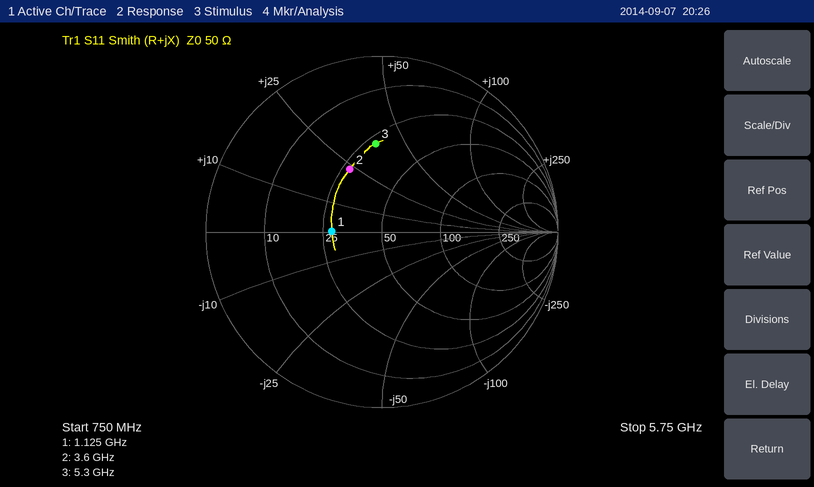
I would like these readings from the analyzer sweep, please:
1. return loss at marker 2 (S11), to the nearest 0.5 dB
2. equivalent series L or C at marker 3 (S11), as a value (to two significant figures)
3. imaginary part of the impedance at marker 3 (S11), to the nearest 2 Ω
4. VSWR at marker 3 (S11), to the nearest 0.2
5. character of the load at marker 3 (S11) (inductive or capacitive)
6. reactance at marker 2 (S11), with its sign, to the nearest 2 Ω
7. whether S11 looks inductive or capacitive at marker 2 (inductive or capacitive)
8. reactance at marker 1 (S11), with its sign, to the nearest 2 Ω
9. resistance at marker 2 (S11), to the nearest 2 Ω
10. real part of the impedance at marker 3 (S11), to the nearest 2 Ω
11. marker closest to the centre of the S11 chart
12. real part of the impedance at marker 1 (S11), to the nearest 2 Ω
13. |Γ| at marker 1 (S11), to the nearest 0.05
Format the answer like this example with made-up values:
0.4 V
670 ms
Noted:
8.0 dB
1.1 nH
+38 Ω
3.0
inductive
+24 Ω
inductive
0 Ω
28 Ω
28 Ω
marker 1
28 Ω
0.30
